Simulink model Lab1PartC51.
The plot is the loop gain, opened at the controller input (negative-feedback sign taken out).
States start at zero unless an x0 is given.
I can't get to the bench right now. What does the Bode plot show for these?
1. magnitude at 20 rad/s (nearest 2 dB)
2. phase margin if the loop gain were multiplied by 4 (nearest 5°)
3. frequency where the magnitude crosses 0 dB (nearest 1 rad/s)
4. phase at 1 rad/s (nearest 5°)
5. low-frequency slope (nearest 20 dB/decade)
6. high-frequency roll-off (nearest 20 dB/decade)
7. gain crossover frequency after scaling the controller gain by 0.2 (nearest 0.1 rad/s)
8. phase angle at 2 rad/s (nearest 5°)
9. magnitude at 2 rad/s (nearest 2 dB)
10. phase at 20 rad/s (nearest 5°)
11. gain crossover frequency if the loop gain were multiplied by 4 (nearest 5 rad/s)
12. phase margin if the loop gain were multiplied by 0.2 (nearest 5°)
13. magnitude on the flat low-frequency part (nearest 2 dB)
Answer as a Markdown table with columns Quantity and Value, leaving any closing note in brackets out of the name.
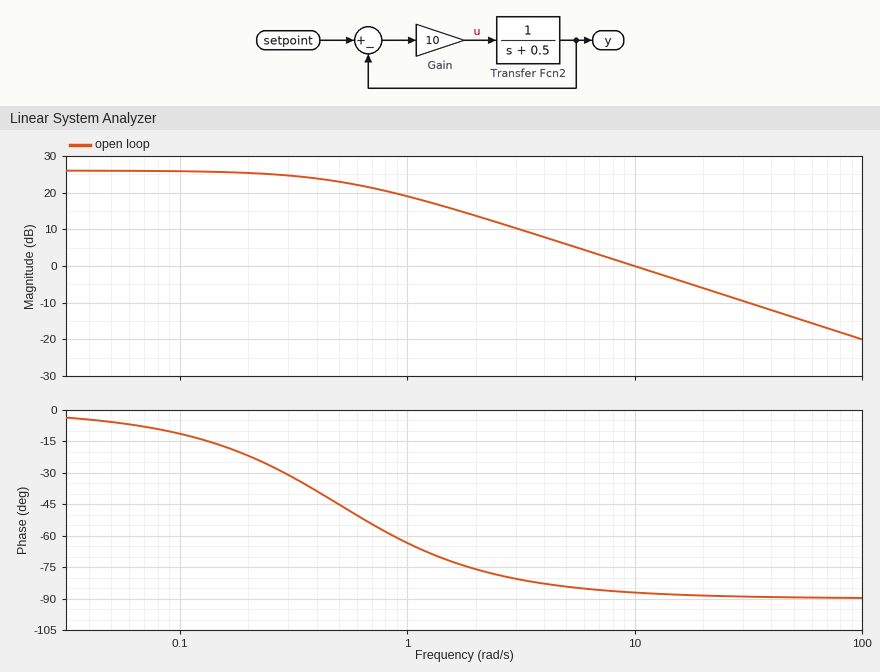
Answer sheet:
| Quantity | Value |
|---|---|
| magnitude at 20 rad/s | -6 dB |
| phase margin if the loop gain were multiplied by 4 | 90° |
| frequency where the magnitude crosses 0 dB | 10 rad/s |
| phase at 1 rad/s | -65° |
| low-frequency slope | 0 dB/decade |
| high-frequency roll-off | -20 dB/decade |
| gain crossover frequency after scaling the controller gain by 0.2 | 1.9 rad/s |
| phase angle at 2 rad/s | -75° |
| magnitude at 2 rad/s | 14 dB |
| phase at 20 rad/s | -90° |
| gain crossover frequency if the loop gain were multiplied by 4 | 40 rad/s |
| phase margin if the loop gain were multiplied by 0.2 | 105° |
| magnitude on the flat low-frequency part | 26 dB |
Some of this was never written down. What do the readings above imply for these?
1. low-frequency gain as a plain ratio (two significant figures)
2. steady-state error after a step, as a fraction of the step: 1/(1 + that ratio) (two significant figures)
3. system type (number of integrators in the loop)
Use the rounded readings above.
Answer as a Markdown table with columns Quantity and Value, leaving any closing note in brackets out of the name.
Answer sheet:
| Quantity | Value |
|---|---|
| low-frequency gain as a plain ratio | 20 |
| steady-state error after a step, as a fraction of the step: 1/(1 + that ratio) | 0.048 |
| system type | 0 |
